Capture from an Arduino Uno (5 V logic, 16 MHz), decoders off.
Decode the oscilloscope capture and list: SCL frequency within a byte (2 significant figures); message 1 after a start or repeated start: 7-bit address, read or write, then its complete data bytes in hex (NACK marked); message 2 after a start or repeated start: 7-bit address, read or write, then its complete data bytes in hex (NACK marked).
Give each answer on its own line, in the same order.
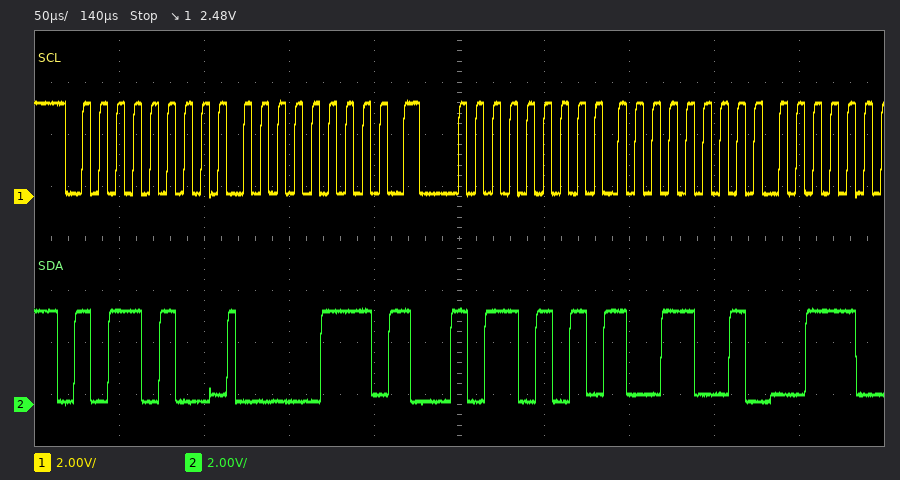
100 kHz
0x5A write: 07
0x5A read: 99
